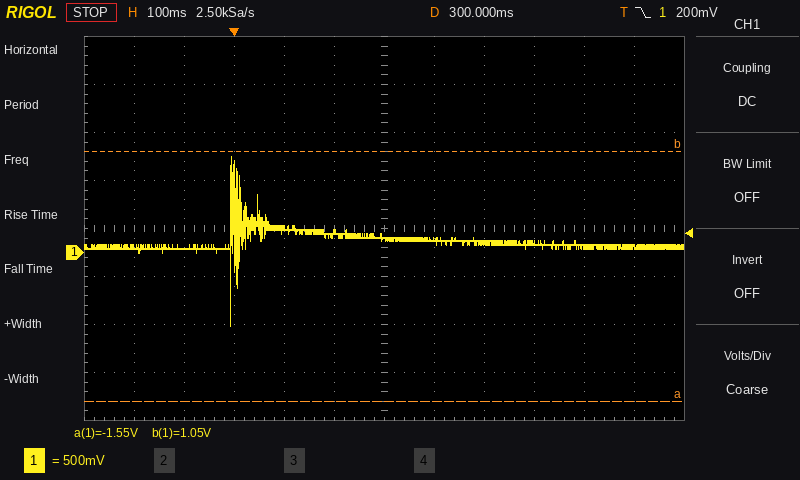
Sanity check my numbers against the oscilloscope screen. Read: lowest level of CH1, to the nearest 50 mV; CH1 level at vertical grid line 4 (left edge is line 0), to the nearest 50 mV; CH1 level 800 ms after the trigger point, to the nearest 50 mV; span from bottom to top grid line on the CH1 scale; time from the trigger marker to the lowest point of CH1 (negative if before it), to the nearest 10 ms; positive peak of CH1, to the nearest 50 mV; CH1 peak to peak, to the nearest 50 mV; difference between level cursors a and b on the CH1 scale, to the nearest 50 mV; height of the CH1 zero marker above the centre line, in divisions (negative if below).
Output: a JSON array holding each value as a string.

["-750 mV", "250 mV", "50 mV", "4 V", "-10 ms", "1.00 V", "1.75 V", "2.60 V", "-0.5 div"]
